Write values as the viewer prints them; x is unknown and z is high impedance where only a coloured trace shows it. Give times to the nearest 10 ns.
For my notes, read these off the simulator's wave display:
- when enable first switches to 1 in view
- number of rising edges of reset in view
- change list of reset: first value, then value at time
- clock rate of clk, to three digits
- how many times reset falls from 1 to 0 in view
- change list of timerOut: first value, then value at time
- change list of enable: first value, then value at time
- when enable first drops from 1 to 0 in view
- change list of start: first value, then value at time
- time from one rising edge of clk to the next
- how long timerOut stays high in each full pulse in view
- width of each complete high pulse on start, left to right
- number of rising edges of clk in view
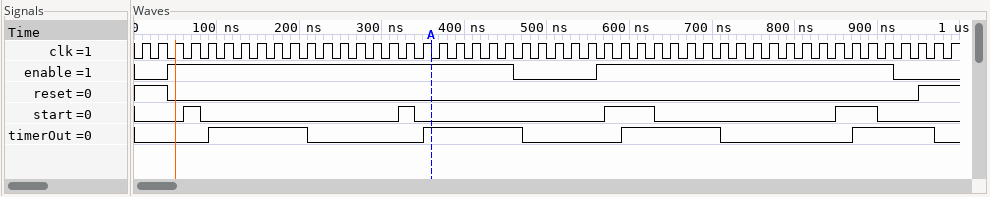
40 ns
1
1, 0 at 40 ns, 1 at 950 ns
50.0 MHz
1
0, 1 at 90 ns, 0 at 210 ns, 1 at 350 ns, 0 at 470 ns, 1 at 590 ns, 0 at 710 ns, 1 at 870 ns, 0 at 970 ns
0, 1 at 40 ns, 0 at 460 ns, 1 at 560 ns, 0 at 920 ns
460 ns
0, 1 at 60 ns, 0 at 80 ns, 1 at 320 ns, 0 at 340 ns, 1 at 570 ns, 0 at 630 ns, 1 at 850 ns, 0 at 900 ns
20 ns
120 ns, 120 ns, 120 ns, 100 ns
20 ns, 20 ns, 60 ns, 50 ns
50
